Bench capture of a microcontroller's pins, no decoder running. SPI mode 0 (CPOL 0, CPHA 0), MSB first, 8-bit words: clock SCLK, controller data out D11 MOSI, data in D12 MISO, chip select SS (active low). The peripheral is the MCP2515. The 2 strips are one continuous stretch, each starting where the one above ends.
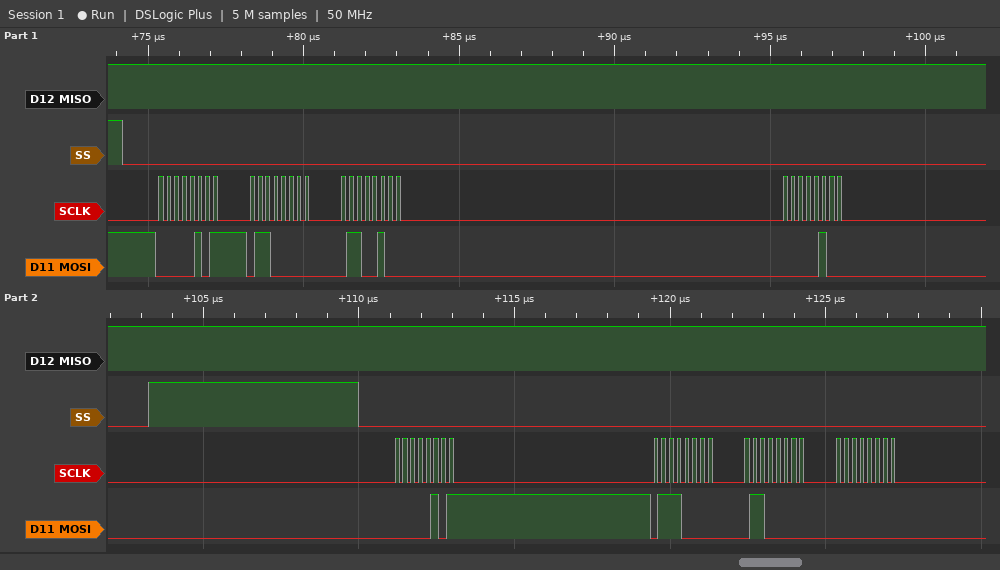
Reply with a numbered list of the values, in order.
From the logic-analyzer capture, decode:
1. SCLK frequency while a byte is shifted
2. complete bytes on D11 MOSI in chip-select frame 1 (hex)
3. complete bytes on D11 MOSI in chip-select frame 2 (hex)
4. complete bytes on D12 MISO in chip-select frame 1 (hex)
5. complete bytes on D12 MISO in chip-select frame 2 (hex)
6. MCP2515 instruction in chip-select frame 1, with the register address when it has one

1. 4 MHz
2. 05 60 64 04
3. 05 70 60 00
4. FF FF FF FF
5. FF FF FF FF
6. BIT MODIFY 0x60
